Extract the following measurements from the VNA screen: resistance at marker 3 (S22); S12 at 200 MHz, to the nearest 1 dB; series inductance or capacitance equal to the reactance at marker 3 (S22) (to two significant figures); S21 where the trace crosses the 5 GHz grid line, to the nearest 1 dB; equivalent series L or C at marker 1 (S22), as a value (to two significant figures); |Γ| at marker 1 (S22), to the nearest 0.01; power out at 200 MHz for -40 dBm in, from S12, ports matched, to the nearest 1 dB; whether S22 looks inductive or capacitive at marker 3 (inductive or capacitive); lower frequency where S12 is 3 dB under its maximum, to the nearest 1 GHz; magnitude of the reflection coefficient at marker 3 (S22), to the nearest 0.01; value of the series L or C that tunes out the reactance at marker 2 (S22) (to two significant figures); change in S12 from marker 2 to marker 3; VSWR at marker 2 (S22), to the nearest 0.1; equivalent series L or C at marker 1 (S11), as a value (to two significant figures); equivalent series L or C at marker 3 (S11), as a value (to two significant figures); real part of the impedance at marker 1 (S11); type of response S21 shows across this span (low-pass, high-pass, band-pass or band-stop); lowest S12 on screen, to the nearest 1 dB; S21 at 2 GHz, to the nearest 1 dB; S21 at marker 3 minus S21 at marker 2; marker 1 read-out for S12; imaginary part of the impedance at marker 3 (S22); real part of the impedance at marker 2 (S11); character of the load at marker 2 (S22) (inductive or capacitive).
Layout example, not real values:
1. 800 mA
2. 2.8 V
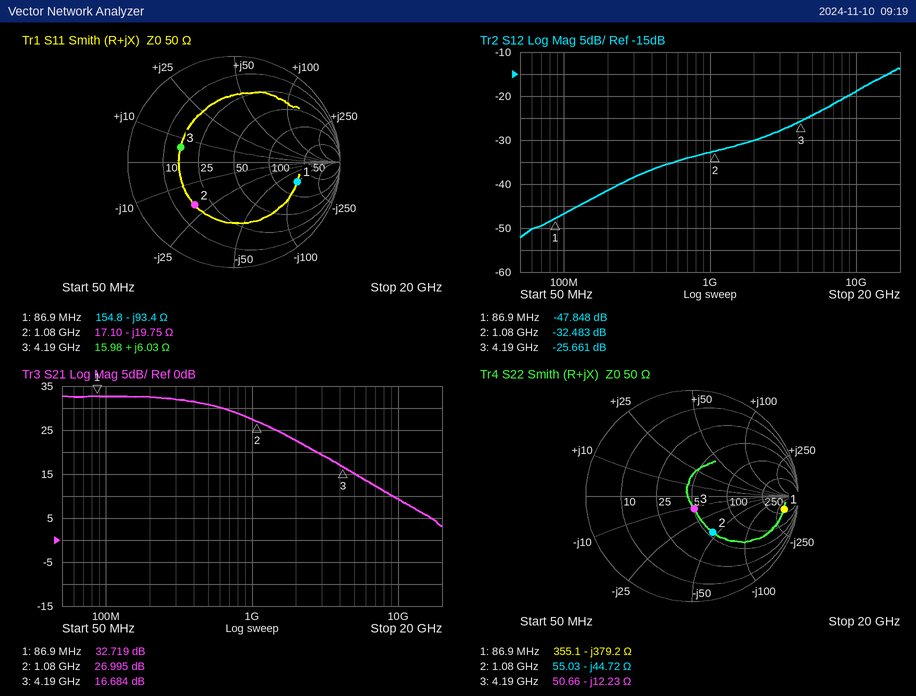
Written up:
1. 50.66 Ω
2. -41 dB
3. 3.1 pF
4. 15 dB
5. 4.8 pF
6. 0.88
7. -81 dBm
8. capacitive
9. 13 GHz
10. 0.12
11. 6.6 nH
12. 6.822 dB
13. 2.3
14. 20 pF
15. 230 pH
16. 154.8 Ω
17. low-pass
18. -52 dB
19. 23 dB
20. -10.311 dB
21. -47.848 dB
22. -12.23 Ω
23. 17.10 Ω
24. capacitive
